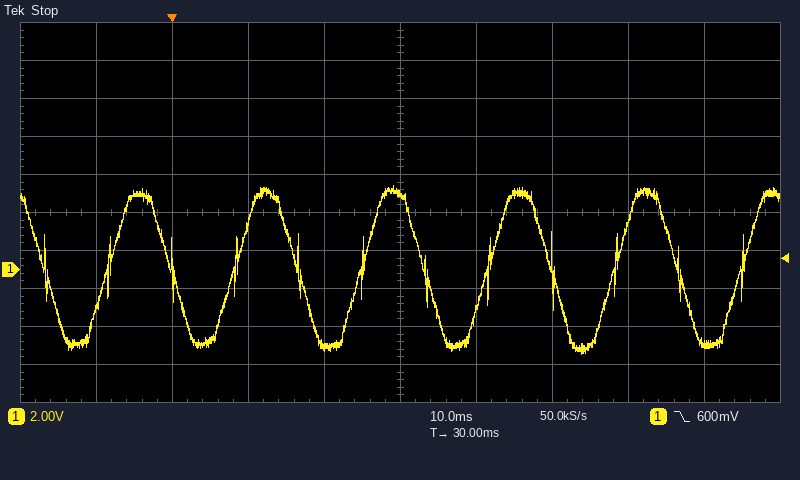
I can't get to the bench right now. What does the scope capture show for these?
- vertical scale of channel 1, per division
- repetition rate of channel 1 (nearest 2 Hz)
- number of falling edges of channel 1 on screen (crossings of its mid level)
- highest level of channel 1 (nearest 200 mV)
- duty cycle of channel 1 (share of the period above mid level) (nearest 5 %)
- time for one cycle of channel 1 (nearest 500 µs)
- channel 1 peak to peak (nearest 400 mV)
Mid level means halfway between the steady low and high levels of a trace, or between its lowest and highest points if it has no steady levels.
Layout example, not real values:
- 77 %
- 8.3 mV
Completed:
- 2 V
- 60 Hz
- 6
- 4.4 V
- 50 %
- 16.5 ms
- 8.8 V
